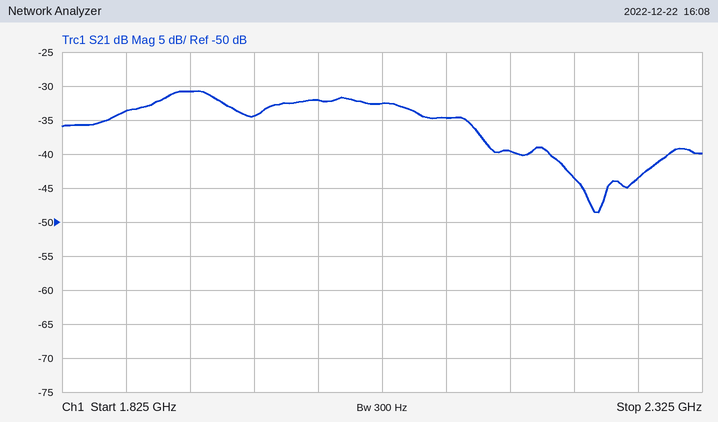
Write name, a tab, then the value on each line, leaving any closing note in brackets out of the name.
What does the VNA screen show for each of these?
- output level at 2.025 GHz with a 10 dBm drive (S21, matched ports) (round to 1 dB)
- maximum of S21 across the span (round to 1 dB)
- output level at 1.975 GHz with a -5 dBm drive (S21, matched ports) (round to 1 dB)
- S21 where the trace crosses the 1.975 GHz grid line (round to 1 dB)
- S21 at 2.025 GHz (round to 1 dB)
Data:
output level at 2.025 GHz with a 10 dBm drive (S21, matched ports)	-22 dBm
maximum of S21 across the span	-31 dB
output level at 1.975 GHz with a -5 dBm drive (S21, matched ports)	-39 dBm
S21 where the trace crosses the 1.975 GHz grid line	-34 dB
S21 at 2.025 GHz	-32 dB
